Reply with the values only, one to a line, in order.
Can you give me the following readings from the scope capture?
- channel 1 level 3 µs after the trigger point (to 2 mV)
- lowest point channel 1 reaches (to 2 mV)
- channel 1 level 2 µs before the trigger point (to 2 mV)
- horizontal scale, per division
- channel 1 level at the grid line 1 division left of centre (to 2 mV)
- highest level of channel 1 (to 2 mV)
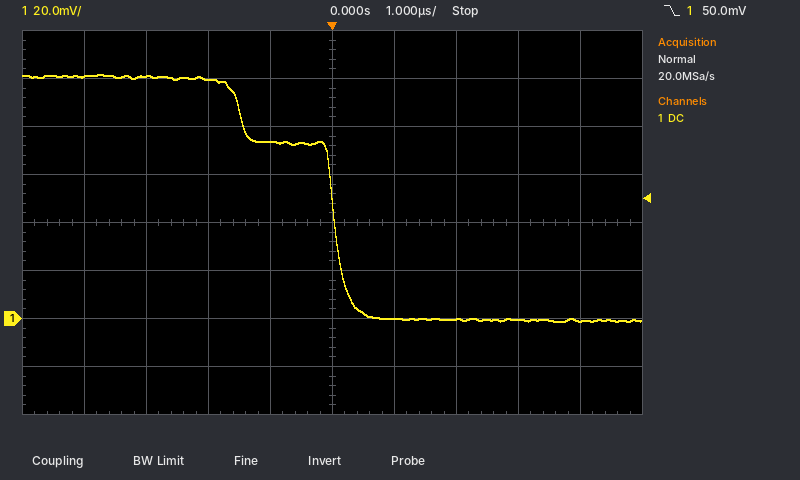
0 mV
-2 mV
100 mV
1 µs
74 mV
102 mV
